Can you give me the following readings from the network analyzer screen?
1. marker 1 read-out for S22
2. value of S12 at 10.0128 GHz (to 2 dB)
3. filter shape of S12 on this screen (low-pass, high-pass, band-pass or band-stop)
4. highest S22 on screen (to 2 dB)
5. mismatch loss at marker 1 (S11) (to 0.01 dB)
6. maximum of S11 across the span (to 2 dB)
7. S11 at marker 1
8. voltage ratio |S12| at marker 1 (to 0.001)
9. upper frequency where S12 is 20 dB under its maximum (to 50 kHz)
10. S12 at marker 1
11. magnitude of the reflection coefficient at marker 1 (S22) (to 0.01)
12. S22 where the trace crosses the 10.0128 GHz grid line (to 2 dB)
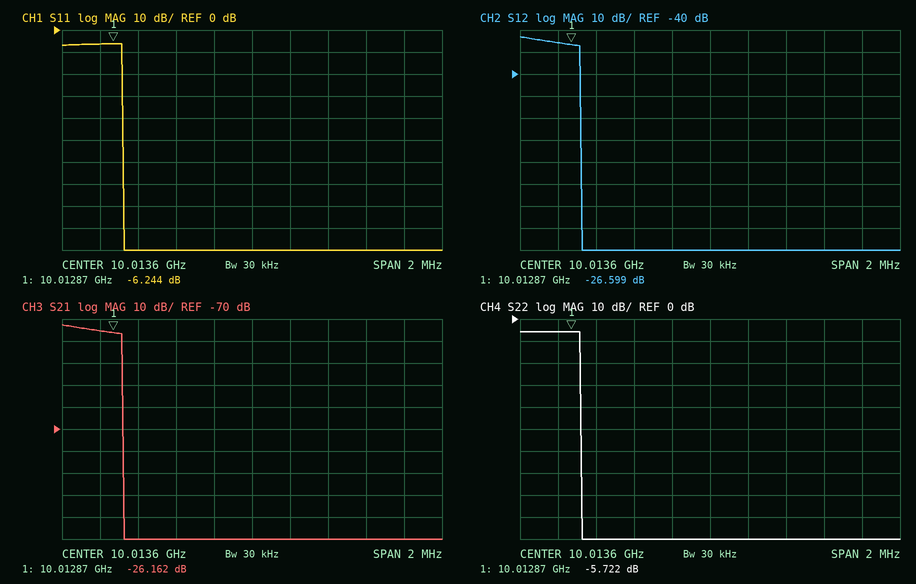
-5.722 dB
-26 dB
low-pass
-6 dB
1.18 dB
-6 dB
-6.244 dB
0.047
10.01290 GHz
-26.599 dB
0.52
-6 dB
